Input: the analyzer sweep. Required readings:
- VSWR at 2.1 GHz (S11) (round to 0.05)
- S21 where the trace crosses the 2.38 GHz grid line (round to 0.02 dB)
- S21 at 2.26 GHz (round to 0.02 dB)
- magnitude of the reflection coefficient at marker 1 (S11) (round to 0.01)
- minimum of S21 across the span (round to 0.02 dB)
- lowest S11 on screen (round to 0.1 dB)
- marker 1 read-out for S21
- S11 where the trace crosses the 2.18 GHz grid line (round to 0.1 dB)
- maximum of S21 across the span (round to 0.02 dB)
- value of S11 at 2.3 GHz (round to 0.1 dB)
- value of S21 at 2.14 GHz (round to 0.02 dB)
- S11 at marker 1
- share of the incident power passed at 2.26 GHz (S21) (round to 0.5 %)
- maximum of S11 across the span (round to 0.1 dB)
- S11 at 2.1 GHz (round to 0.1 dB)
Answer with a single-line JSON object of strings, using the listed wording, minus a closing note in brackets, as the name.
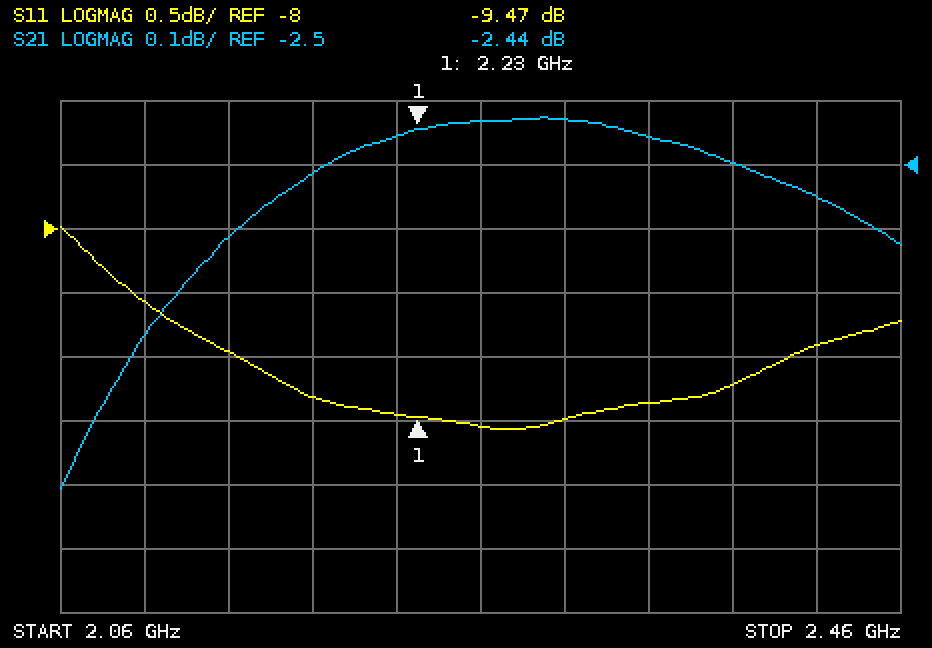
{"VSWR at 2.1 GHz (S11)": "2.20", "S21 where the trace crosses the 2.38 GHz grid line": "-2.50 dB", "S21 at 2.26 GHz": "-2.44 dB", "magnitude of the reflection coefficient at marker 1 (S11)": "0.34", "minimum of S21 across the span": "-3.00 dB", "lowest S11 on screen": "-9.6 dB", "marker 1 read-out for S21": "-2.44 dB", "S11 where the trace crosses the 2.18 GHz grid line": "-9.3 dB", "maximum of S21 across the span": "-2.42 dB", "value of S11 at 2.3 GHz": "-9.5 dB", "value of S21 at 2.14 GHz": "-2.62 dB", "S11 at marker 1": "-9.47 dB", "share of the incident power passed at 2.26 GHz (S21)": "57.0 %", "maximum of S11 across the span": "-8.0 dB", "S11 at 2.1 GHz": "-8.6 dB"}
